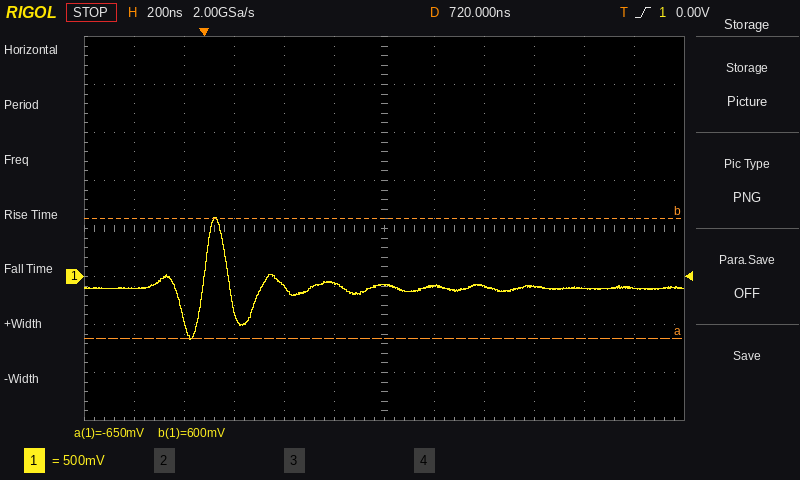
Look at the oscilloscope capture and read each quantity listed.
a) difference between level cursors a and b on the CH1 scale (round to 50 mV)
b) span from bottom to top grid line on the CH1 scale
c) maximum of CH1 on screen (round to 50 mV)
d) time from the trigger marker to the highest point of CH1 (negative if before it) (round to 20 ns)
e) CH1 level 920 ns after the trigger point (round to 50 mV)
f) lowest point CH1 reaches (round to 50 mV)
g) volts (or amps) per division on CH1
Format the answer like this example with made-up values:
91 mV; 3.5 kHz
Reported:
1.25 V; 4 V; 600 mV; +40 ns; -100 mV; -650 mV; 500 mV
